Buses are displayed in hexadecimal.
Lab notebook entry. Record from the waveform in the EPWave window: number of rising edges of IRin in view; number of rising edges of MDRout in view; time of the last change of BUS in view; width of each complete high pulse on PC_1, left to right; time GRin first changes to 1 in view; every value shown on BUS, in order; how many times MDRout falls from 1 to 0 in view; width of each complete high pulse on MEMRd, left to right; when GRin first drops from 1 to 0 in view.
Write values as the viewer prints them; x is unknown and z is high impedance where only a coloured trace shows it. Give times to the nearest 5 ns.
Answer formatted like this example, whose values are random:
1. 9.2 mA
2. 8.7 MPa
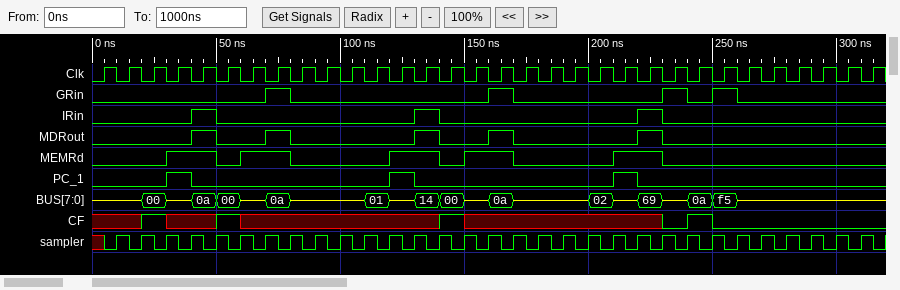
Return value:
1. 3
2. 5
3. 260 ns
4. 10 ns, 10 ns, 10 ns
5. 70 ns
6. z, 00, z, 0a, 00, z, 0a, z, 01, z, 14, 00, z, 0a, z, 02, z, 69, z, 0a, f5, z
7. 5
8. 20 ns, 20 ns, 20 ns, 20 ns, 20 ns
9. 80 ns
